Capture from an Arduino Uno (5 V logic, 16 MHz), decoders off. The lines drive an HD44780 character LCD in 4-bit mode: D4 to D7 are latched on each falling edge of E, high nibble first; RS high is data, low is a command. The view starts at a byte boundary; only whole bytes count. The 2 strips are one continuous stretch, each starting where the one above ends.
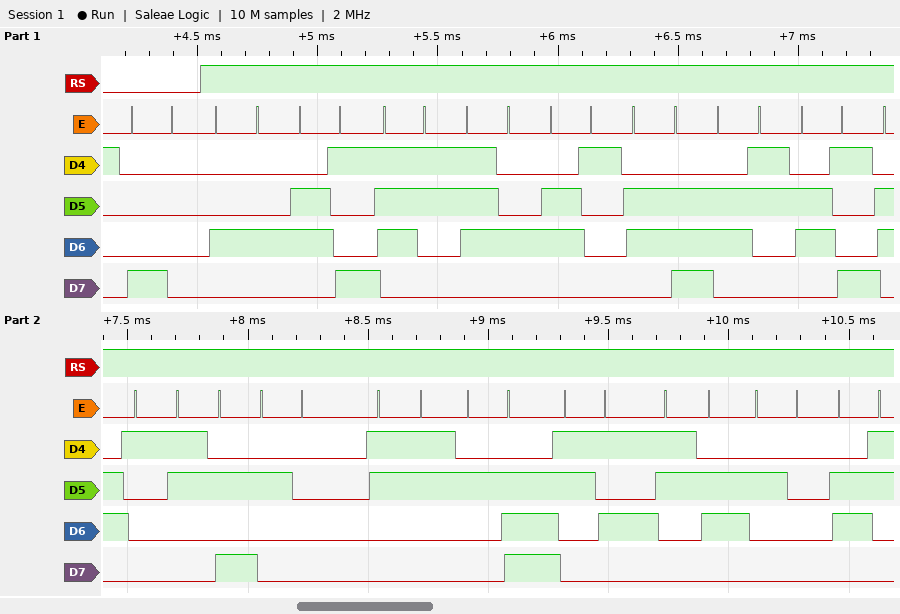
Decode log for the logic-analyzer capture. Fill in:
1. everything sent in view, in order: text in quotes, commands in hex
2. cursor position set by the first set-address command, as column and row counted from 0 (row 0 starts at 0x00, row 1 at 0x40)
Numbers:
0x80 "Distancia: 3.56 c"
column 0, row 0
